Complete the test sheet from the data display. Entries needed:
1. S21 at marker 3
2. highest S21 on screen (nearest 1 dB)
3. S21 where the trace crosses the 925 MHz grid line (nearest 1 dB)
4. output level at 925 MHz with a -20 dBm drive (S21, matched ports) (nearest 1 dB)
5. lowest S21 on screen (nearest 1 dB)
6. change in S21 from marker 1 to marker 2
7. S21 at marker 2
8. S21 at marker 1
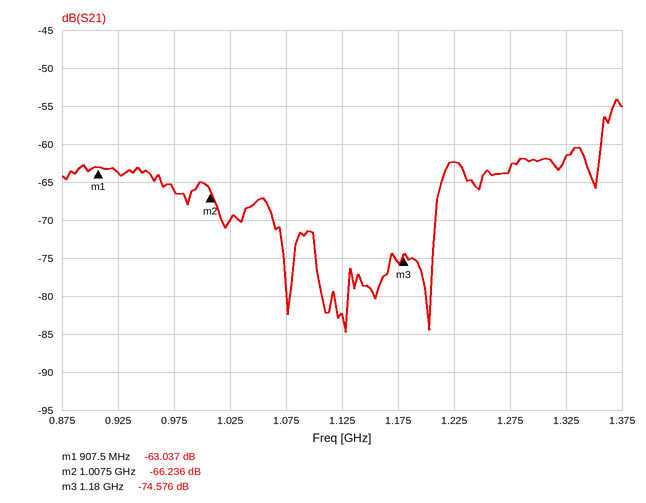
-74.576 dB
-54 dB
-64 dB
-84 dBm
-85 dB
-3.199 dB
-66.236 dB
-63.037 dB
